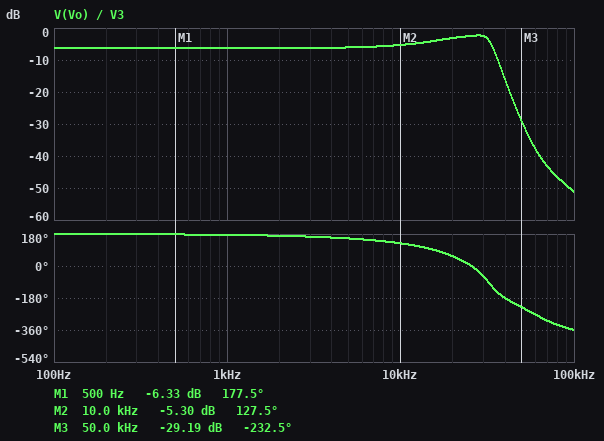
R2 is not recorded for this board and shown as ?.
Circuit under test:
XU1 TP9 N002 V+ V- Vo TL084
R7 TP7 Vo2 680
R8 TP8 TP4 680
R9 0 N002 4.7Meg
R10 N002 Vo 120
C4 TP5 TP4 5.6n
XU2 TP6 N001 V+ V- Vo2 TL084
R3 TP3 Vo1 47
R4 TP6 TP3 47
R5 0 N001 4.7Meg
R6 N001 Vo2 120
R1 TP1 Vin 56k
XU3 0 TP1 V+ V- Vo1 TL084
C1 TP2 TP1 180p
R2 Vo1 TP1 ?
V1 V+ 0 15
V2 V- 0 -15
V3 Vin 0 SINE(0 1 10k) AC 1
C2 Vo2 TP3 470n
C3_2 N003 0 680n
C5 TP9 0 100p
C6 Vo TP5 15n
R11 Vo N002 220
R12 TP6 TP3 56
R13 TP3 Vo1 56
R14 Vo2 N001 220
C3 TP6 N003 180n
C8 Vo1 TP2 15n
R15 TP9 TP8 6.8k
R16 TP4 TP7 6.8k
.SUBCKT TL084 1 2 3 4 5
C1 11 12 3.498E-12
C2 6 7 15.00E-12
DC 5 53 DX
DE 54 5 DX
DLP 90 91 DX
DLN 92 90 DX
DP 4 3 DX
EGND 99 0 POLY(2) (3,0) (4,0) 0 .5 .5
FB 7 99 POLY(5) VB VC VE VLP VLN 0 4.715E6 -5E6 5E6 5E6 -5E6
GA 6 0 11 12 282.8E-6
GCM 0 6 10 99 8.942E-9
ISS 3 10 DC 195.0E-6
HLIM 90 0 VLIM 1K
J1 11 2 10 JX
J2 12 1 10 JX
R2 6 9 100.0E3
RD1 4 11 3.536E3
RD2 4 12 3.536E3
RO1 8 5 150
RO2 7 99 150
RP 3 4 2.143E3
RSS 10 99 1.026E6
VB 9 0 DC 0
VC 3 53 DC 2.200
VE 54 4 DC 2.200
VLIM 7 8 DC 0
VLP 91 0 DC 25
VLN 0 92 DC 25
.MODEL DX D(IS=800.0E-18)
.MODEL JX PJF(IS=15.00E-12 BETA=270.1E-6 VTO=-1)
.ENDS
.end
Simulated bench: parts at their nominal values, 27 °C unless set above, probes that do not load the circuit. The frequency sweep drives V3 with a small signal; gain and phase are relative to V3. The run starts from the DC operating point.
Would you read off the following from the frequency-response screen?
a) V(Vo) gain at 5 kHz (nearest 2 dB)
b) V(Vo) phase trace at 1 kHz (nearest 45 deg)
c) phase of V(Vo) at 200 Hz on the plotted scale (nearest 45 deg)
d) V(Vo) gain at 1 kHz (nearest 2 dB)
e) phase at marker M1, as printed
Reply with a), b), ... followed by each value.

a) -6 dB
b) 180 deg
c) 180 deg
d) -6 dB
e) 177.5 deg
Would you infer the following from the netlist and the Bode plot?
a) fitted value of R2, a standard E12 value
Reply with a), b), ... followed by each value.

a) 27 kΩ
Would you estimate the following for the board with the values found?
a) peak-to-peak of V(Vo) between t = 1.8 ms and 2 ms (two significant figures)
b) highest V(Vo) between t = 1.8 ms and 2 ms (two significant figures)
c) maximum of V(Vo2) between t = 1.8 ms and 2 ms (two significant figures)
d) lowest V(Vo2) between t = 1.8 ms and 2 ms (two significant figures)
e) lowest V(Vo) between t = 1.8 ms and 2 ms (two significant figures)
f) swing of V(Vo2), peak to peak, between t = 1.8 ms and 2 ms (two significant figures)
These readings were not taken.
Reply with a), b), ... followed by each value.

a) 1.1 V
b) 540 mV
c) 490 mV
d) -490 mV
e) -540 mV
f) 990 mV
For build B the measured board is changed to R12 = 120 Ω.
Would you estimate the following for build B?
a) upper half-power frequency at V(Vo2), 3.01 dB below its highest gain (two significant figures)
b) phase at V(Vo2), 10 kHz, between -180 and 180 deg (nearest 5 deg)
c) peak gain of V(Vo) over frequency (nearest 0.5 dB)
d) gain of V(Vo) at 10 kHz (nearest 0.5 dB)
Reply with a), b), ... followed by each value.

a) 22 kHz
b) 130 deg
c) -4.0 dB
d) -5.0 dB
